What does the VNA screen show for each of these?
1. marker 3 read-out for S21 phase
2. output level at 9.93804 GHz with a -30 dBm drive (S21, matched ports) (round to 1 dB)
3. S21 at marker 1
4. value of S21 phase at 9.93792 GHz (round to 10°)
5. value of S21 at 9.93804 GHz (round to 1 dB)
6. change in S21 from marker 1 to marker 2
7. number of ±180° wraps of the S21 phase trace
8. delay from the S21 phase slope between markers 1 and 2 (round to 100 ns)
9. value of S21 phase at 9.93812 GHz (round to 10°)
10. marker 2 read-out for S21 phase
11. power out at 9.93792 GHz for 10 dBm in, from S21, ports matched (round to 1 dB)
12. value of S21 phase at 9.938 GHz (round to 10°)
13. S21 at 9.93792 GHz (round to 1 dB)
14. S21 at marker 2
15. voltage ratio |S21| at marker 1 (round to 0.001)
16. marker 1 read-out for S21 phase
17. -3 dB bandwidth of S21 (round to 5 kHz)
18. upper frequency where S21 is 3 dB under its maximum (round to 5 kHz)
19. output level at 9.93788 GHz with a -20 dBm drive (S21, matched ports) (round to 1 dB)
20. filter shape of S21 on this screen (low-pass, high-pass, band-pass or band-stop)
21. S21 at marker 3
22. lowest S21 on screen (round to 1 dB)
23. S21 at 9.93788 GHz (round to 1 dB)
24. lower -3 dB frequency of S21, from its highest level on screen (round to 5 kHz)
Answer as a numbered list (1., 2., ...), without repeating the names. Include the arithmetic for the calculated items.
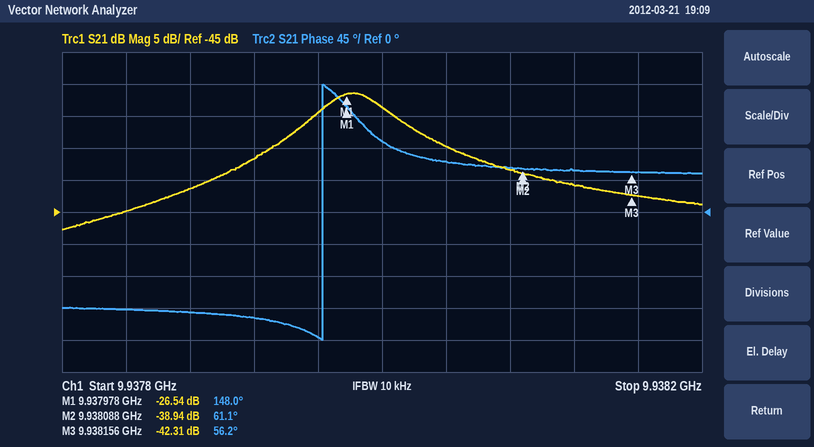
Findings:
1. 56.2°
2. -30 dBm + (-35 dB) = -65 dBm
3. -26.54 dB
4. -150°
5. -35 dB
6. -38.94 − (-26.54) = -12.40 dB
7. 1
8. −(61.1° − (148°))/(360° × 110 kHz) ≈ 2.2 µs
9. 60°
10. 61.1°
11. 10 dBm + (-37 dB) = -27 dBm
12. 100°
13. -37 dB
14. -38.94 dB
15. 10^(-26.54/20) ≈ 0.047
16. 148.0°
17. 9.938005 GHz − 9.937960 GHz = 45 kHz
18. 9.938005 GHz
19. -20 dBm + (-41 dB) = -61 dBm
20. band-pass
21. -42.31 dB
22. -48 dB
23. -41 dB
24. 9.937960 GHz
